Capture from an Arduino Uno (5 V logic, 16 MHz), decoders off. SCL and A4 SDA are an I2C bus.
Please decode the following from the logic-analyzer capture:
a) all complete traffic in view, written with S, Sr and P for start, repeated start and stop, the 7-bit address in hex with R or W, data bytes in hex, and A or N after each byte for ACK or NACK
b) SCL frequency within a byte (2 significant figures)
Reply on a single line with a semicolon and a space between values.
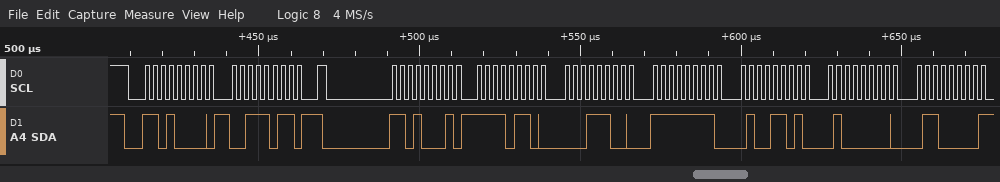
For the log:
S 68W A 3B A Sr 68R A F6 A 1C A FF A 4D A 40 A 60 N; 400 kHz
